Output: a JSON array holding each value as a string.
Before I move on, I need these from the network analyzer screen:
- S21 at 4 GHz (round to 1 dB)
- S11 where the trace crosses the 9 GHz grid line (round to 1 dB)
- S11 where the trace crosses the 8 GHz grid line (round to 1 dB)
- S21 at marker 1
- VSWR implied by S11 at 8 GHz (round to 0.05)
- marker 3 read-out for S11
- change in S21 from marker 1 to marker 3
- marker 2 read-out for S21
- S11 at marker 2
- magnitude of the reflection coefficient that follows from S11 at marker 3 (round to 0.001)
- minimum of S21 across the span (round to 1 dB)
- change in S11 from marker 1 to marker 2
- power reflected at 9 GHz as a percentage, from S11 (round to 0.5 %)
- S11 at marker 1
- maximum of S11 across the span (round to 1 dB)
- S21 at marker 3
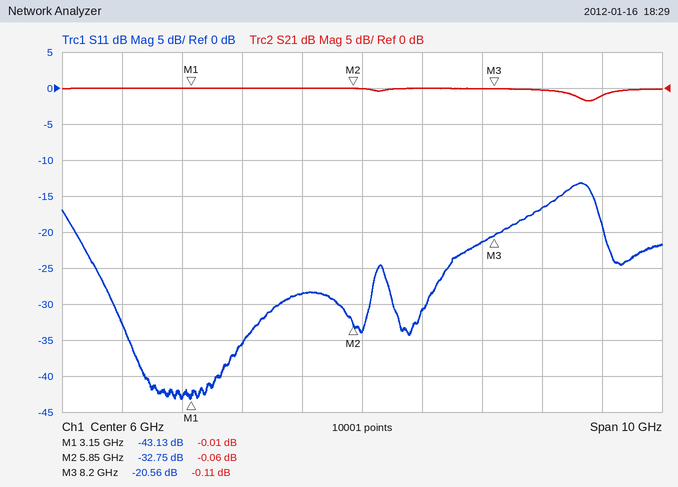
["0 dB", "-17 dB", "-21 dB", "-0.01 dB", "1.20", "-20.56 dB", "-0.10 dB", "-0.06 dB", "-32.75 dB", "0.094", "-2 dB", "10.38 dB", "2.0 %", "-43.13 dB", "-13 dB", "-0.11 dB"]
